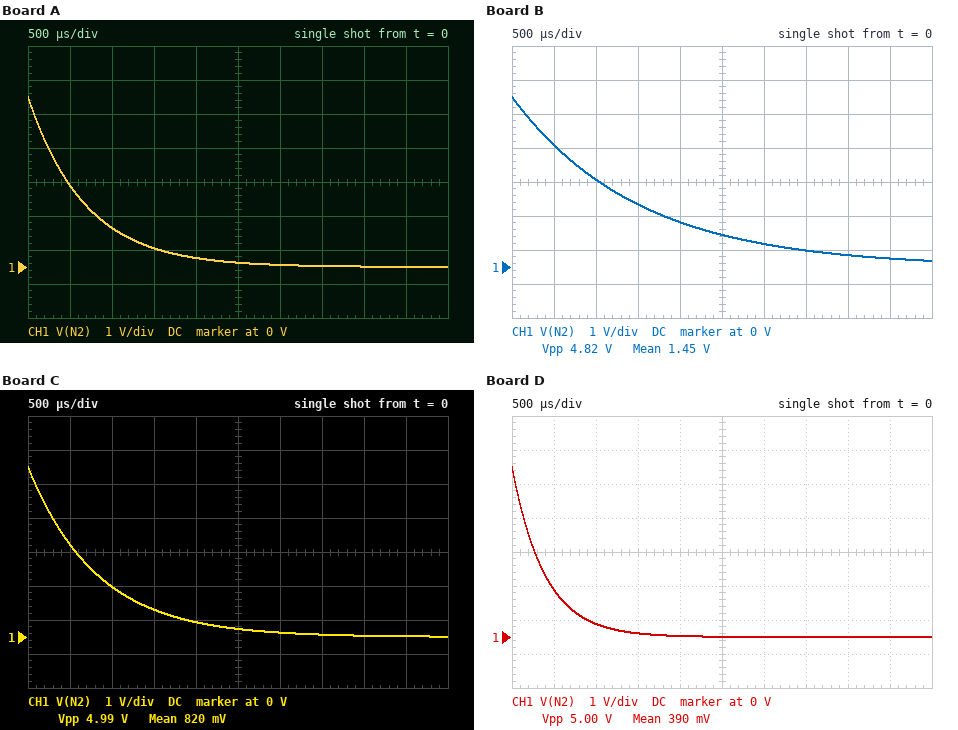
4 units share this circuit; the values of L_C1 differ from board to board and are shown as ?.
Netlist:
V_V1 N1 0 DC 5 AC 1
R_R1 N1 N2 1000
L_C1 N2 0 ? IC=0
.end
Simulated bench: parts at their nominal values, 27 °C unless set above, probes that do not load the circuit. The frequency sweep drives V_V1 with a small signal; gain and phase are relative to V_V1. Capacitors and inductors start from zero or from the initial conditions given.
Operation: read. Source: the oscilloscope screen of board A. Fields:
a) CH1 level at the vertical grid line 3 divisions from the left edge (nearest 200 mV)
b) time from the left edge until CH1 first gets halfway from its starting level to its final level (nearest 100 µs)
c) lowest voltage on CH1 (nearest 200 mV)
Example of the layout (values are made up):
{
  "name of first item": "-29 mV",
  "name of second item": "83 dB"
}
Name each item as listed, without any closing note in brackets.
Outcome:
{
  "CH1 level at the vertical grid line 3 divisions from the left edge": "600 mV",
  "time from the left edge until CH1 first gets halfway from its starting level to its final level": "500 µs",
  "lowest voltage on CH1": "0 V"
}
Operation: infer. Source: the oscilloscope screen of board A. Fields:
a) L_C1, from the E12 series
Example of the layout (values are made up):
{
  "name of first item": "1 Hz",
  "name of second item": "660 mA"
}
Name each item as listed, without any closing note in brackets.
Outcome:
{
  "L_C1, from the E12 series": "680 mH"
}
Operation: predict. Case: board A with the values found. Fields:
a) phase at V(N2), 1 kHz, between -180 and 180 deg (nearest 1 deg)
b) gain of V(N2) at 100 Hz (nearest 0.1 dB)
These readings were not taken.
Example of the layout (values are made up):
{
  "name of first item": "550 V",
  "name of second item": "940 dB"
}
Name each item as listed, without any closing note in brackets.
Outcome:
{
  "phase at V(N2), 1 kHz, between -180 and 180 deg": "13 deg",
  "gain of V(N2) at 100 Hz": "-8.1 dB"
}
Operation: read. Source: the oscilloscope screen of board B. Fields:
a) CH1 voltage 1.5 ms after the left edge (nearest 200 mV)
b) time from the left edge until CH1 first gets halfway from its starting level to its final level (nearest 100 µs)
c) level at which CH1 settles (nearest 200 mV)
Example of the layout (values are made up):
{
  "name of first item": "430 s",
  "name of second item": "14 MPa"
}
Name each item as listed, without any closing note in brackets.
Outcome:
{
  "CH1 voltage 1.5 ms after the left edge": "1.8 V",
  "time from the left edge until CH1 first gets halfway from its starting level to its final level": "1.0 ms",
  "level at which CH1 settles": "200 mV"
}
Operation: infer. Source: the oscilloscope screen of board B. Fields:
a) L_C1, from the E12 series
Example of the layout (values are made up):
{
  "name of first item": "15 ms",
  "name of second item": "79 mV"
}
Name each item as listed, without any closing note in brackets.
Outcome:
{
  "L_C1, from the E12 series": "1.5 H"
}
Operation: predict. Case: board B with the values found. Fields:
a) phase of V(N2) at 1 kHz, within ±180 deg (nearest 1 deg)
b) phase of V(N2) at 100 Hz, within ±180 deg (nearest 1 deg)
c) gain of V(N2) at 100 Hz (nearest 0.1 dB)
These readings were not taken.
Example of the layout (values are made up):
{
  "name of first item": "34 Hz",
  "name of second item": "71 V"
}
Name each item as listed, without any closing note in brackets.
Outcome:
{
  "phase of V(N2) at 1 kHz, within ±180 deg": "6 deg",
  "phase of V(N2) at 100 Hz, within ±180 deg": "47 deg",
  "gain of V(N2) at 100 Hz": "-3.3 dB"
}
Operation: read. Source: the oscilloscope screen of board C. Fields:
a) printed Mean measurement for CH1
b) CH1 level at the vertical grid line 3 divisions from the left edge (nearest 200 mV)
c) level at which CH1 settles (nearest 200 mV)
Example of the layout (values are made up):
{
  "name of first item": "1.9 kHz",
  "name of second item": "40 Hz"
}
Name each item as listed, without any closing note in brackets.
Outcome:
{
  "printed Mean measurement for CH1": "820 mV",
  "CH1 level at the vertical grid line 3 divisions from the left edge": "800 mV",
  "level at which CH1 settles": "0 V"
}
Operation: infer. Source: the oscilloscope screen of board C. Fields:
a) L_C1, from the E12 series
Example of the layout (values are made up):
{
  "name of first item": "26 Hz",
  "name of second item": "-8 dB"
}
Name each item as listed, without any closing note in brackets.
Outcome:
{
  "L_C1, from the E12 series": "820 mH"
}
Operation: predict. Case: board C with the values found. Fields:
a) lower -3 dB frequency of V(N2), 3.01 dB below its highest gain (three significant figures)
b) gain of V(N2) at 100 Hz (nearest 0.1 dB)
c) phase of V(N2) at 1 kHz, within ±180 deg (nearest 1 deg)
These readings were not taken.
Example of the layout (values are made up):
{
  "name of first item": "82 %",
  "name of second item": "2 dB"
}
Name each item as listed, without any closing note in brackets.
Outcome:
{
  "lower -3 dB frequency of V(N2), 3.01 dB below its highest gain": "194 Hz",
  "gain of V(N2) at 100 Hz": "-6.8 dB",
  "phase of V(N2) at 1 kHz, within ±180 deg": "11 deg"
}
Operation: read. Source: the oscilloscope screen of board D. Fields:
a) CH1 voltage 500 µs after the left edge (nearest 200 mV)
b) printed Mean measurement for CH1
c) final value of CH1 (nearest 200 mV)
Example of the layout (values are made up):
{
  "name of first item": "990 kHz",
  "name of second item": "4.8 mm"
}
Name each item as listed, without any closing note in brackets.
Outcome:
{
  "CH1 voltage 500 µs after the left edge": "1.4 V",
  "printed Mean measurement for CH1": "390 mV",
  "final value of CH1": "0 V"
}
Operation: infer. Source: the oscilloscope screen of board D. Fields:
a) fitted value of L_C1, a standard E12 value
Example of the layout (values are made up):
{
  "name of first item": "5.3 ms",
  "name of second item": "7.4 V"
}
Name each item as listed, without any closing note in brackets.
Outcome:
{
  "fitted value of L_C1, a standard E12 value": "390 mH"
}
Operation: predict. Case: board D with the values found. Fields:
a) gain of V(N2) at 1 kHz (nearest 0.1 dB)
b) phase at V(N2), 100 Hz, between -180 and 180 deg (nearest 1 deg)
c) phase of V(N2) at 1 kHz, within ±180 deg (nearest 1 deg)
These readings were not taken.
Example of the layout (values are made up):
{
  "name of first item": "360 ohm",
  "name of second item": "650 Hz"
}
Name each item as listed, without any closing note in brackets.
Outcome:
{
  "gain of V(N2) at 1 kHz": "-0.7 dB",
  "phase at V(N2), 100 Hz, between -180 and 180 deg": "76 deg",
  "phase of V(N2) at 1 kHz, within ±180 deg": "22 deg"
}
